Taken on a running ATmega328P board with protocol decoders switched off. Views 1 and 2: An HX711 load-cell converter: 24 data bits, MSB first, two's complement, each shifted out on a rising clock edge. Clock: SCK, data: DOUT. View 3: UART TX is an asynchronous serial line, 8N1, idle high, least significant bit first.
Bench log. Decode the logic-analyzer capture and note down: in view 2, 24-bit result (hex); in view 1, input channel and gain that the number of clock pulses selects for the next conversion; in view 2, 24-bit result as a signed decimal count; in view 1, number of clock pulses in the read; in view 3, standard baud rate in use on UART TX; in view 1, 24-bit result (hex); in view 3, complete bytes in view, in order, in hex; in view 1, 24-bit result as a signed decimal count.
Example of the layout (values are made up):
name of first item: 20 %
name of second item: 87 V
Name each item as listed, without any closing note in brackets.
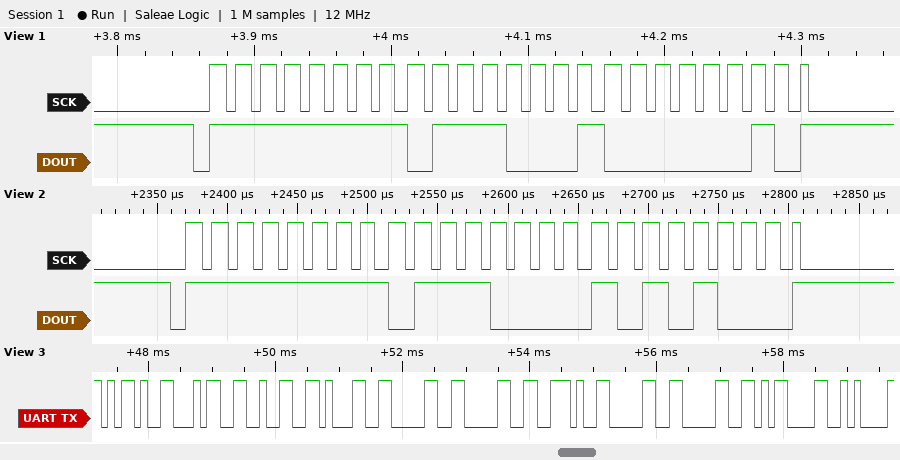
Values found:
in view 2, 24-bit result: 0xFF70A8
in view 1, input channel and gain that the number of clock pulses selects for the next conversion: channel A, gain 128
in view 2, 24-bit result as a signed decimal count: -36696
in view 1, number of clock pulses in the read: 25
in view 3, standard baud rate in use on UART TX: 9600 baud
in view 1, 24-bit result: 0xFF7102
in view 3, complete bytes in view, in order, in hex: 2D 34 32 31 30 30 2E 30 30 0D 0A
in view 1, 24-bit result as a signed decimal count: -36606
